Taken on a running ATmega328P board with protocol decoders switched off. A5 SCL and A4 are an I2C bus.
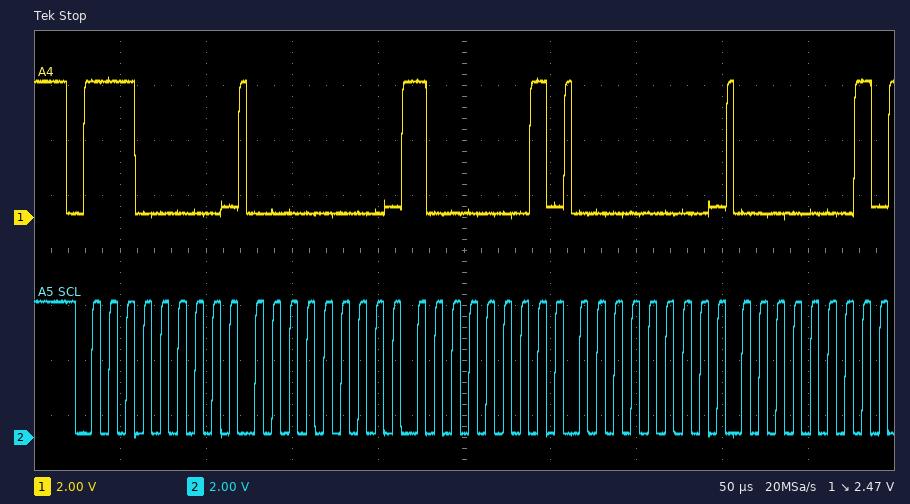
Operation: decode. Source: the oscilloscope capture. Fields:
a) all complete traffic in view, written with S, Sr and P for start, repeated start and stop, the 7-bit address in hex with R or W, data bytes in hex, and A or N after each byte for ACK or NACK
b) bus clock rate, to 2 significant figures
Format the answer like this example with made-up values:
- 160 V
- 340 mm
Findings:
- S 70W A 00 A 81 A 00 A 01 A
- 100 kHz
